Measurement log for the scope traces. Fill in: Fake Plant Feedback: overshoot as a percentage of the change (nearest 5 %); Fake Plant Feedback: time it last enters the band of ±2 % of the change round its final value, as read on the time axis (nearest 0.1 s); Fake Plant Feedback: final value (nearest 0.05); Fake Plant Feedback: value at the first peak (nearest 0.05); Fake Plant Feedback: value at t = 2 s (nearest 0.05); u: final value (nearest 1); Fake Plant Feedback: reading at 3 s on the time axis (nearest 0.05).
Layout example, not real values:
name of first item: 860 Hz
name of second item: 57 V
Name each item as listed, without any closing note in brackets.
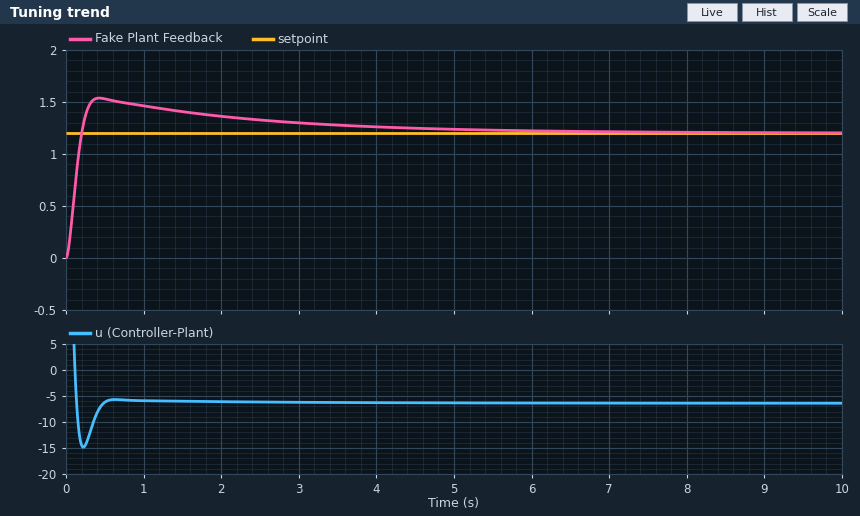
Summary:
Fake Plant Feedback: overshoot as a percentage of the change: 30 %
Fake Plant Feedback: time it last enters the band of ±2 % of the change round its final value, as read on the time axis: 5.9 s
Fake Plant Feedback: final value: 1.20
Fake Plant Feedback: value at the first peak: 1.55
Fake Plant Feedback: value at t = 2 s: 1.35
u: final value: -6
Fake Plant Feedback: reading at 3 s on the time axis: 1.30
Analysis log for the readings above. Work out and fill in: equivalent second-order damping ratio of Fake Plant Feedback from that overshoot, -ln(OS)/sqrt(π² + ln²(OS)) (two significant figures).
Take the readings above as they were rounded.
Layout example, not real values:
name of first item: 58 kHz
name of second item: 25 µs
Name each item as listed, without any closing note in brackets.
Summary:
equivalent second-order damping ratio of Fake Plant Feedback from that overshoot, -ln(OS)/sqrt(π² + ln²(OS)): 0.36
